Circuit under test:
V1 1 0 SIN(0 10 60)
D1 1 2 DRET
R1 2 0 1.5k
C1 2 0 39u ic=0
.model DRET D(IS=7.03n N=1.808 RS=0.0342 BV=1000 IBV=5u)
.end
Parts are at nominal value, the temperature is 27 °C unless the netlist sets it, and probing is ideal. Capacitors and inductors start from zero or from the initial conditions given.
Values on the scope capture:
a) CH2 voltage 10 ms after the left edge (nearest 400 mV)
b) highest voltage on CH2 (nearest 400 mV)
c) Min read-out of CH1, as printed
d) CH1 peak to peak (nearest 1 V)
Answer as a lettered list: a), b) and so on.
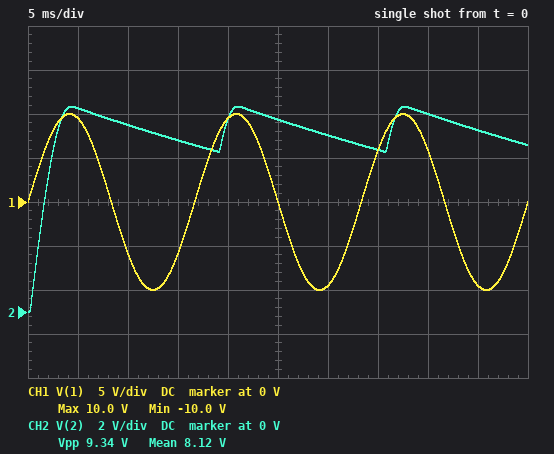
a) 8.4 V
b) 9.2 V
c) -10.0 V
d) 20 V
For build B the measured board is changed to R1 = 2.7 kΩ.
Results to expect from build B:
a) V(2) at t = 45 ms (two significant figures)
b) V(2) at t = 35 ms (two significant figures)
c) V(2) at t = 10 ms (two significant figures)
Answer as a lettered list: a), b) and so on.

a) 8.7 V
b) 8.2 V
c) 8.9 V
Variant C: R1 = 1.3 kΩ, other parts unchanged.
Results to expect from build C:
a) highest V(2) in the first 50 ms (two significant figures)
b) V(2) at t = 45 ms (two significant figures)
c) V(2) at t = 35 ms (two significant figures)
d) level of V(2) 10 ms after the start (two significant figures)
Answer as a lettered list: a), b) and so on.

a) 9.3 V
b) 8.1 V
c) 7.1 V
d) 8.4 V
